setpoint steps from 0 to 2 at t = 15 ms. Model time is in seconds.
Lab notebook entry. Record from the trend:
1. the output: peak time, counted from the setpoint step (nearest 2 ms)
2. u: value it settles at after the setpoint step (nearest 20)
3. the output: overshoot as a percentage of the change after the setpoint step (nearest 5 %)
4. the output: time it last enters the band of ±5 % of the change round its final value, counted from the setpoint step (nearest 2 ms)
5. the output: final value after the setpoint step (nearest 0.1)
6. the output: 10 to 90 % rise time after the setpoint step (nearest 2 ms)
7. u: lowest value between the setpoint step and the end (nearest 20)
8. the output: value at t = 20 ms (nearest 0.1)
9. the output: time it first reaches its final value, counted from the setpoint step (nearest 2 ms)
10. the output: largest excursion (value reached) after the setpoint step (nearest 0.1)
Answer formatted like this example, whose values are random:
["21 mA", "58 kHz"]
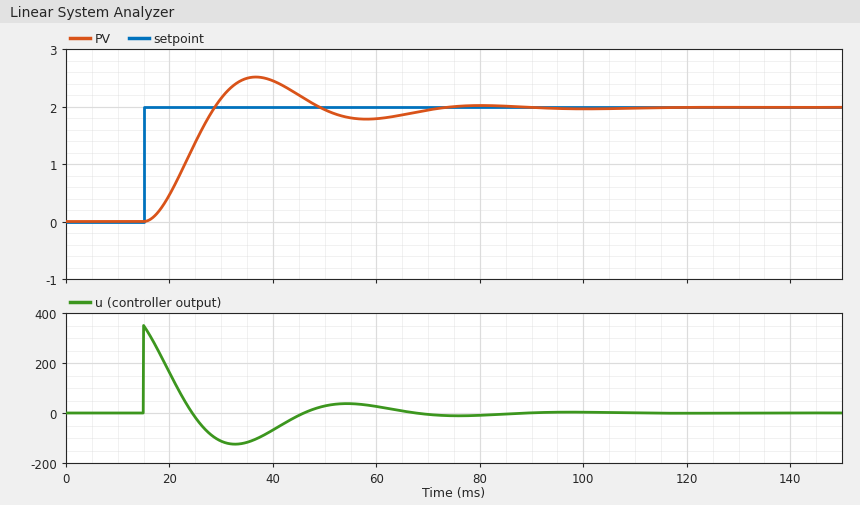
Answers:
["22 ms", "0", "25 %", "52 ms", "2.0", "10 ms", "-120", "0.5", "14 ms", "2.5"]
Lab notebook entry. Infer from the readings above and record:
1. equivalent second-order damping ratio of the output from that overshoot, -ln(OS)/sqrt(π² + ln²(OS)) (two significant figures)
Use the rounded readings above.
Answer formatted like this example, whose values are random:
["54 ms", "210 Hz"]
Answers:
["0.40"]
